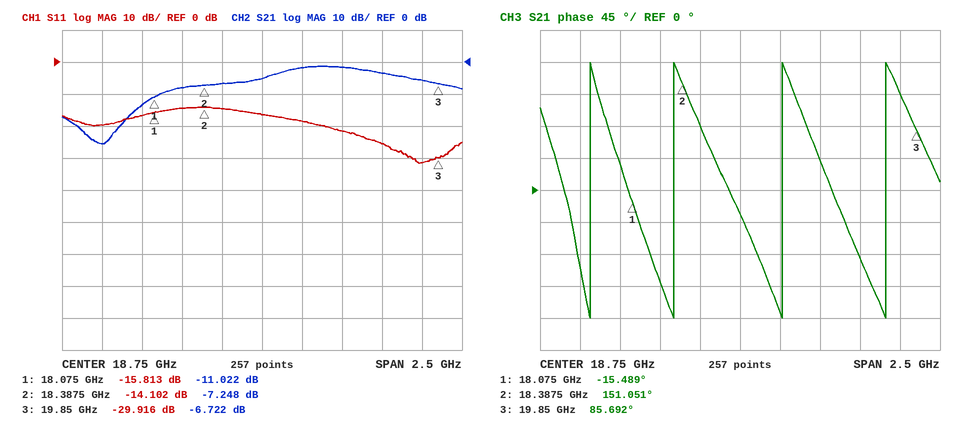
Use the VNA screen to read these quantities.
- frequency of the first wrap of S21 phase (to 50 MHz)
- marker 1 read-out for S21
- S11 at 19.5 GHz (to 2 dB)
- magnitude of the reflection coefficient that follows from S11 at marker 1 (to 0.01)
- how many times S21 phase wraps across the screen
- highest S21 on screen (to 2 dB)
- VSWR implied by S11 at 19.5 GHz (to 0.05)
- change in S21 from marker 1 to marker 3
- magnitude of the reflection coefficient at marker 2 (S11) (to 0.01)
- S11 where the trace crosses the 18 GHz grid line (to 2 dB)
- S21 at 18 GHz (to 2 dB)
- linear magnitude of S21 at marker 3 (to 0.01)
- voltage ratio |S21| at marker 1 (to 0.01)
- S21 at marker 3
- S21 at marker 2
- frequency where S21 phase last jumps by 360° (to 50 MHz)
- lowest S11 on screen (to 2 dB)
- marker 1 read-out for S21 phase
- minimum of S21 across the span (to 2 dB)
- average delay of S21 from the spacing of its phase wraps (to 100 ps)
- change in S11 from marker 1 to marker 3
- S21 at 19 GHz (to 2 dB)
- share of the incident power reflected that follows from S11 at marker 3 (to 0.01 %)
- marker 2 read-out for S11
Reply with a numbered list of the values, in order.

1. 17.80 GHz
2. -11.022 dB
3. -26 dB
4. 0.16
5. 4
6. -2 dB
7. 1.10
8. 4.300 dB
9. 0.20
10. -16 dB
11. -14 dB
12. 0.46
13. 0.28
14. -6.722 dB
15. -7.248 dB
16. 19.65 GHz
17. -32 dB
18. -15.489°
19. -26 dB
20. 1.6 ns
21. -14.103 dB
22. -2 dB
23. 0.10 %
24. -14.102 dB
